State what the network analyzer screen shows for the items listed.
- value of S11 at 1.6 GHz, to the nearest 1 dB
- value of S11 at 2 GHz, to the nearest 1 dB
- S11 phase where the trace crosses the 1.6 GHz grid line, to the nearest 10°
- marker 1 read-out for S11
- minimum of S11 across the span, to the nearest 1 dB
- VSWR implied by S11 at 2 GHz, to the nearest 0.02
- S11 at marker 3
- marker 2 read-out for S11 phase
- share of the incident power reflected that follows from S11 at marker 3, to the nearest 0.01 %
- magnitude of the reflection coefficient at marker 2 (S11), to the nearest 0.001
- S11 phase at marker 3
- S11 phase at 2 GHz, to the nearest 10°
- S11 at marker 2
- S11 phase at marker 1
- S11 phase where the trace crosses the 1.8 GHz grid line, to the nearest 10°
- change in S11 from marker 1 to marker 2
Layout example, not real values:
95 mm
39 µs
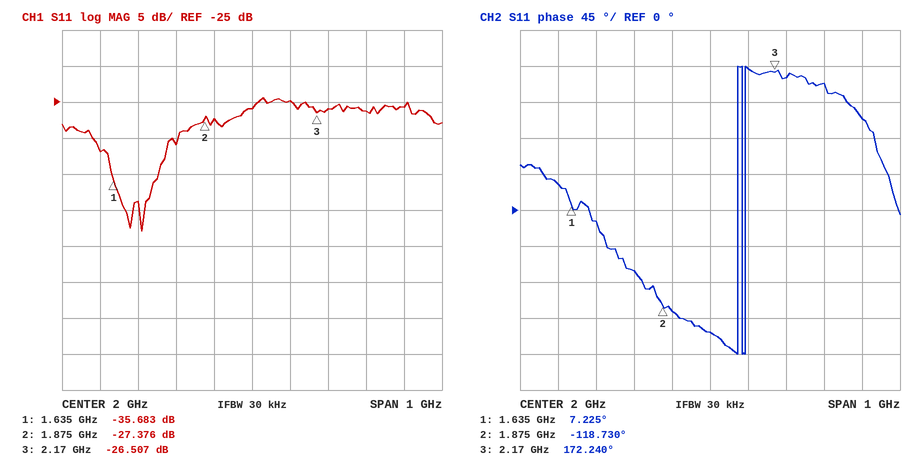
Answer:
-32 dB
-26 dB
30°
-35.683 dB
-43 dB
1.10
-26.507 dB
-118.730°
0.22 %
0.043
172.240°
-150°
-27.376 dB
7.225°
-80°
8.307 dB
